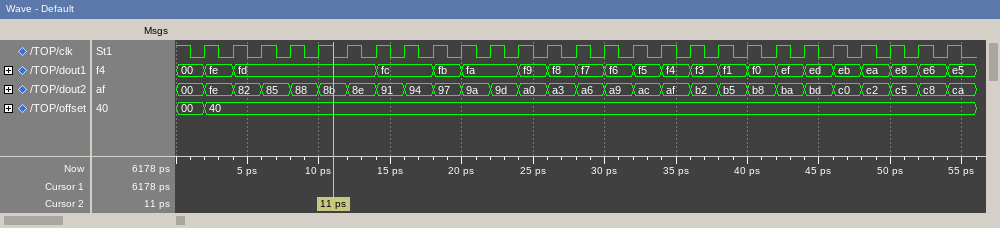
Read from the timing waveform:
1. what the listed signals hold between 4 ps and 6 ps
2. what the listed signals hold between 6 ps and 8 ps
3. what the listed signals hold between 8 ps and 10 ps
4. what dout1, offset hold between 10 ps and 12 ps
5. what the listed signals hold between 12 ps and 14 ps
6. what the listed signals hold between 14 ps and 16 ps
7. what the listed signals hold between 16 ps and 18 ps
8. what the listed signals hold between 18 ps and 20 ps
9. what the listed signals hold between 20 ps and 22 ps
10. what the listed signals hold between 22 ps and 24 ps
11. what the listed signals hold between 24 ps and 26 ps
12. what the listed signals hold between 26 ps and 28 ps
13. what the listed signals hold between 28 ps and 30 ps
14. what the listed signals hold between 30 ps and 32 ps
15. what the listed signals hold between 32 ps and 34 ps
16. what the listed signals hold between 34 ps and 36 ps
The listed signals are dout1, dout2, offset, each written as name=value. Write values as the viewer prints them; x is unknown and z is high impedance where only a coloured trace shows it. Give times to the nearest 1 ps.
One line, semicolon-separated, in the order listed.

dout1=fd, dout2=82, offset=40; dout1=fd, dout2=85, offset=40; dout1=fd, dout2=88, offset=40; dout1=fd, offset=40; dout1=fd, dout2=8e, offset=40; dout1=fc, dout2=91, offset=40; dout1=fc, dout2=94, offset=40; dout1=fb, dout2=97, offset=40; dout1=fa, dout2=9a, offset=40; dout1=fa, dout2=9d, offset=40; dout1=f9, dout2=a0, offset=40; dout1=f8, dout2=a3, offset=40; dout1=f7, dout2=a6, offset=40; dout1=f6, dout2=a9, offset=40; dout1=f5, dout2=ac, offset=40; dout1=f4, dout2=af, offset=40
